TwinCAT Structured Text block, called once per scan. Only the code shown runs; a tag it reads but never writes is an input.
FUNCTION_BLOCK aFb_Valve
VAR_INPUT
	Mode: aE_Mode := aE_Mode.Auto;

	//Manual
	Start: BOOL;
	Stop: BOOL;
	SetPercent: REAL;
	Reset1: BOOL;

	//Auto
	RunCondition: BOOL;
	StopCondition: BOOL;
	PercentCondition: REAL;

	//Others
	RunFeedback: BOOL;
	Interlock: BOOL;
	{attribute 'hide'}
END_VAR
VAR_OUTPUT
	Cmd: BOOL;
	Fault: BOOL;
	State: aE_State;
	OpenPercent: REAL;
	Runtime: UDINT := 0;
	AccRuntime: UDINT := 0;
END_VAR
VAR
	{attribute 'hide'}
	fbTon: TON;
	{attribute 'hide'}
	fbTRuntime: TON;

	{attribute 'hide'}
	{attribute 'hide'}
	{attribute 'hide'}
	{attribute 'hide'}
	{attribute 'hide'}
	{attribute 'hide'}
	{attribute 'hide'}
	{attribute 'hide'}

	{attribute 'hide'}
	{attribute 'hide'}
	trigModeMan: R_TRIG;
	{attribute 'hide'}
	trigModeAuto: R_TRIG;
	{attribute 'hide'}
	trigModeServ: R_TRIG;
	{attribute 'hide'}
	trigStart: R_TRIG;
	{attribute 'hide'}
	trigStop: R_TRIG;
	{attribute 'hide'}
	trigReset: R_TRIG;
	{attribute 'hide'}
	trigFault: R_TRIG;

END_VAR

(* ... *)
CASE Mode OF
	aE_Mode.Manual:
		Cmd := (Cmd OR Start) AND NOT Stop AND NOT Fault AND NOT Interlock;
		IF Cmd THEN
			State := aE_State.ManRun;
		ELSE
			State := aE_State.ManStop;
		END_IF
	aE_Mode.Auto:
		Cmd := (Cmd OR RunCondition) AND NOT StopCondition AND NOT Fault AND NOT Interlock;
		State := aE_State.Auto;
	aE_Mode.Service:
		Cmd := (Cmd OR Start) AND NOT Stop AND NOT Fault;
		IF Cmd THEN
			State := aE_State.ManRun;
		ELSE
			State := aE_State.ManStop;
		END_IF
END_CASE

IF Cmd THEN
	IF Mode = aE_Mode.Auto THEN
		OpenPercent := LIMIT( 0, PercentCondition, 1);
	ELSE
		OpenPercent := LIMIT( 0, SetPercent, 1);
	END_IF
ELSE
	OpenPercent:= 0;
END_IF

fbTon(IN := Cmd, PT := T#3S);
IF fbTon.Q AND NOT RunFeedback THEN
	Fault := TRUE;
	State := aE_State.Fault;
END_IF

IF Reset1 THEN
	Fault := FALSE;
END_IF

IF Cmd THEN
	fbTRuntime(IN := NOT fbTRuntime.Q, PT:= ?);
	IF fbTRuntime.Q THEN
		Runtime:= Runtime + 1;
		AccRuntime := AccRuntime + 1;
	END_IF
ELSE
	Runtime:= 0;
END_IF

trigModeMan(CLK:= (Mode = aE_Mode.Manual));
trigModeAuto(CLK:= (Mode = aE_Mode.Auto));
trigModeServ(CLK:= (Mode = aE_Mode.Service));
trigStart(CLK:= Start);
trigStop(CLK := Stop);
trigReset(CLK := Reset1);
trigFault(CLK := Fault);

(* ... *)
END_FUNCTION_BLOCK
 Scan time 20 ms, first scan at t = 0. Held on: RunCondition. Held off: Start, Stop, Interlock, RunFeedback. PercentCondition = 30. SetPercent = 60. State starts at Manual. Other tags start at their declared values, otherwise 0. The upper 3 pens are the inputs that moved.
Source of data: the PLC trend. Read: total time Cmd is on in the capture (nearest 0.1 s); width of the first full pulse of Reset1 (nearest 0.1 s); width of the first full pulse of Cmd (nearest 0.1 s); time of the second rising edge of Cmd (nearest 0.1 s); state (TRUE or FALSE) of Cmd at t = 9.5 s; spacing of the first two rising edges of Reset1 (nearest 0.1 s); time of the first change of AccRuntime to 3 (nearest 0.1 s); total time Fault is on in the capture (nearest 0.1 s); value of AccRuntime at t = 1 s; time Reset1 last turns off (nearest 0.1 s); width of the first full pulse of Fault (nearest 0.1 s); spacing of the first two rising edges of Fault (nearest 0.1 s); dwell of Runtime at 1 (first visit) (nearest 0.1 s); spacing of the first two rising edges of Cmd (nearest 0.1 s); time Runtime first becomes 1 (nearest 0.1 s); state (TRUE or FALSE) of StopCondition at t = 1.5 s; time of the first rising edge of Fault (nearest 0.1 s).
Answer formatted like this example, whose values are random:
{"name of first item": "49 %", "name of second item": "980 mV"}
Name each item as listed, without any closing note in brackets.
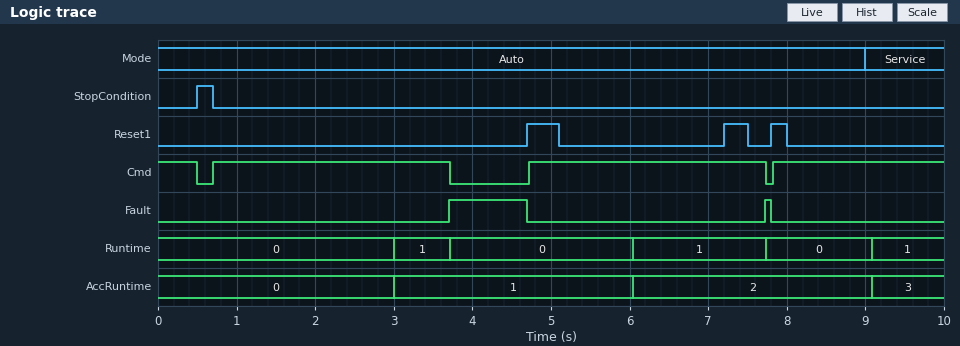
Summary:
{"total time Cmd is on in the capture": "8.7 s", "width of the first full pulse of Reset1": "0.4 s", "width of the first full pulse of Cmd": "3.0 s", "time of the second rising edge of Cmd": "4.7 s", "state (TRUE or FALSE) of Cmd at t = 9.5 s": "TRUE", "spacing of the first two rising edges of Reset1": "2.5 s", "time of the first change of AccRuntime to 3": "9.1 s", "total time Fault is on in the capture": "1.1 s", "value of AccRuntime at t = 1 s": "0", "time Reset1 last turns off": "8.0 s", "width of the first full pulse of Fault": "1.0 s", "spacing of the first two rising edges of Fault": "4.0 s", "dwell of Runtime at 1 (first visit)": "0.7 s", "spacing of the first two rising edges of Cmd": "4.0 s", "time Runtime first becomes 1": "3.0 s", "state (TRUE or FALSE) of StopCondition at t = 1.5 s": "FALSE", "time of the first rising edge of Fault": "3.7 s"}
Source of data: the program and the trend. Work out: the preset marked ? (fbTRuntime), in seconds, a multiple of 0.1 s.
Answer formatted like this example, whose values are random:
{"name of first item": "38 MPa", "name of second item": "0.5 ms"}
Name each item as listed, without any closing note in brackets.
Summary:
{"the preset marked ? (fbTRuntime), in seconds, a multiple of 0.1 s": "3.0 s"}
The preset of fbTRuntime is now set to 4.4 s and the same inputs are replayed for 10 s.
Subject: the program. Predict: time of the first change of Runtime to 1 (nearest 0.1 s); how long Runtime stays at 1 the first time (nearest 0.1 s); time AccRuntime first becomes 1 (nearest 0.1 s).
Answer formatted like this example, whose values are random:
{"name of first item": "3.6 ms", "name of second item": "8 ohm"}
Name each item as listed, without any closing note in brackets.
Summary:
{"time of the first change of Runtime to 1": "4.7 s", "how long Runtime stays at 1 the first time": "3.0 s", "time AccRuntime first becomes 1": "4.7 s"}
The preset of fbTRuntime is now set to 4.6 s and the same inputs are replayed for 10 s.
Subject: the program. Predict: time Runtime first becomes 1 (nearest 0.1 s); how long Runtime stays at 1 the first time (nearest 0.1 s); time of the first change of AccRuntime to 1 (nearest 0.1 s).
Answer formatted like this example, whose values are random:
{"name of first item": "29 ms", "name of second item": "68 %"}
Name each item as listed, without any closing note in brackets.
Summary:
{"time Runtime first becomes 1": "4.7 s", "how long Runtime stays at 1 the first time": "3.0 s", "time of the first change of AccRuntime to 1": "4.7 s"}
